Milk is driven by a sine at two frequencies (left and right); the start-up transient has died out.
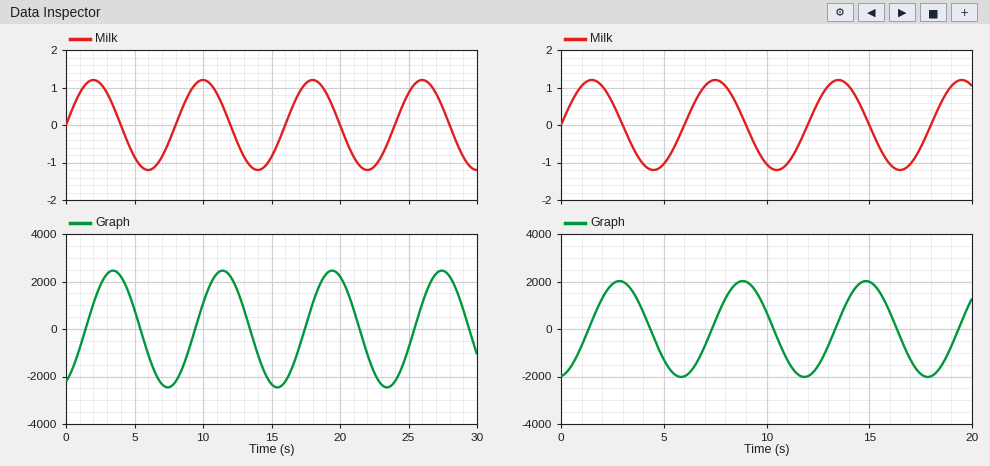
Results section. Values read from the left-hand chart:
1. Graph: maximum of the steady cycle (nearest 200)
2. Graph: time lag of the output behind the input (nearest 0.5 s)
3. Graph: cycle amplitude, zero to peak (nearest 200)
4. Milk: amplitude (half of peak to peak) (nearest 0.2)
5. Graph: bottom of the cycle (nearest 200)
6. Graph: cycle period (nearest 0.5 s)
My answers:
2400
1.5 s
2400
1.2
-2400
8.0 s
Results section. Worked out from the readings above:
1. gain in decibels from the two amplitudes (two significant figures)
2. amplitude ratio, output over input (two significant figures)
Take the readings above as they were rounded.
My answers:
66 dB
2000
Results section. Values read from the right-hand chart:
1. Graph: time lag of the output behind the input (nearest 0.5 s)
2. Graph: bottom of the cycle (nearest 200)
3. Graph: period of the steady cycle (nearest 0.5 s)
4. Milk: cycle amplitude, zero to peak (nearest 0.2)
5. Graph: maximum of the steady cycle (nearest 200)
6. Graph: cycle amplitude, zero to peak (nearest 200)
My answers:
1.5 s
-2000
6.0 s
1.2
2000
2000
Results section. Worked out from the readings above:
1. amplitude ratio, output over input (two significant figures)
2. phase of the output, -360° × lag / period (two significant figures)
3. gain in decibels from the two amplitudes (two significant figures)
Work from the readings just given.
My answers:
1700
-90°
64 dB
